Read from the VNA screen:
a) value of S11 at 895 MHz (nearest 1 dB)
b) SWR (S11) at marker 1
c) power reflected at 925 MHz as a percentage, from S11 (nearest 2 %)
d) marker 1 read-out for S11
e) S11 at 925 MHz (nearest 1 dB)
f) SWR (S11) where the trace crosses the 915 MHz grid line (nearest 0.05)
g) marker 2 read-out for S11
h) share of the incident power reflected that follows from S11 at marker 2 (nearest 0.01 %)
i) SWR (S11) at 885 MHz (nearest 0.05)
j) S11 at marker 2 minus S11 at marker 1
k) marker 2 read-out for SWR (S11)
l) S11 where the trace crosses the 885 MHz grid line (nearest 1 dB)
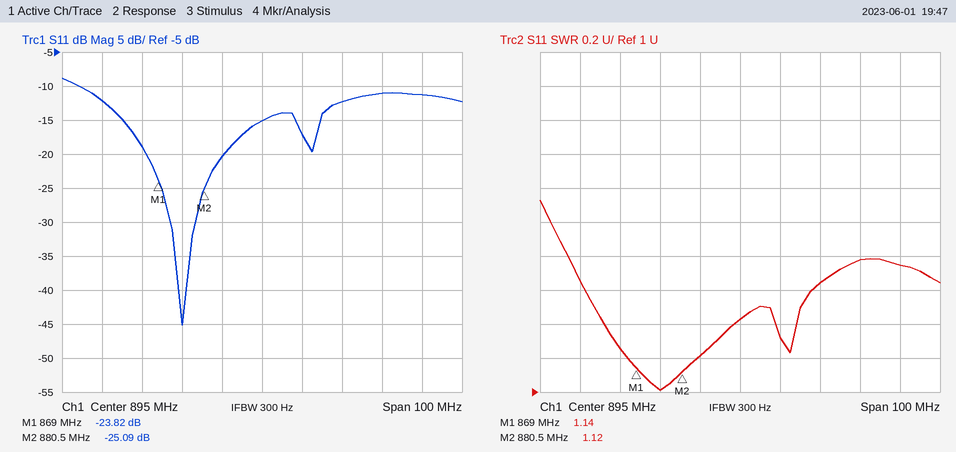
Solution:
-15 dB
1.14
8 %
-23.82 dB
-11 dB
1.65
-25.09 dB
0.31 %
1.20
-1.27 dB
1.12
-20 dB
